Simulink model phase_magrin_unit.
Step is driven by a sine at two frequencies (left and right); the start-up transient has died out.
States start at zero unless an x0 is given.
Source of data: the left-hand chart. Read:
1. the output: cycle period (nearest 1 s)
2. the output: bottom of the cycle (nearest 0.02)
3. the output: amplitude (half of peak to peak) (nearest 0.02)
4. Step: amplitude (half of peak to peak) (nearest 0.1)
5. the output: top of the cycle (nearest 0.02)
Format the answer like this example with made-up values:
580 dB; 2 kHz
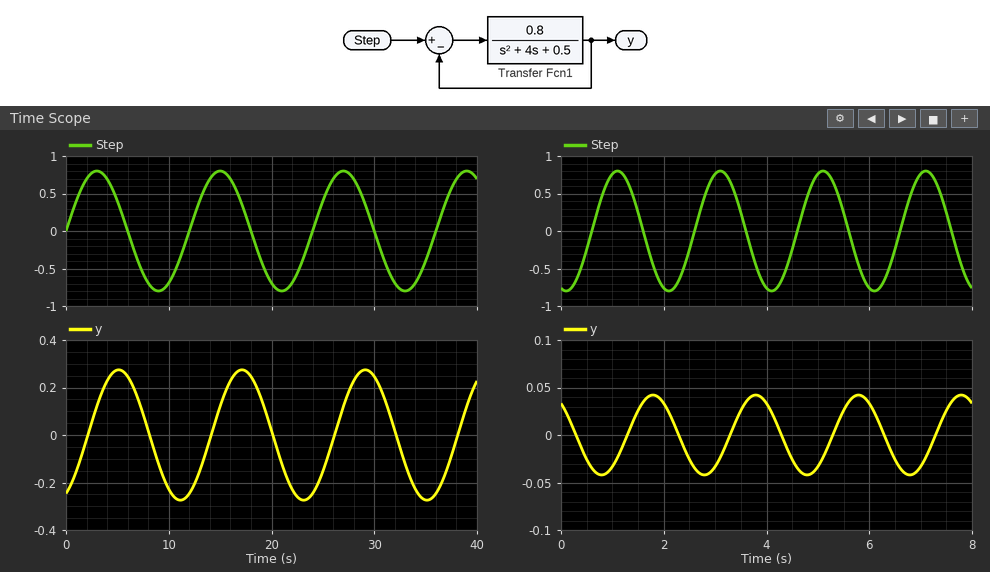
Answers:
12 s; -0.28; 0.28; 0.8; 0.28
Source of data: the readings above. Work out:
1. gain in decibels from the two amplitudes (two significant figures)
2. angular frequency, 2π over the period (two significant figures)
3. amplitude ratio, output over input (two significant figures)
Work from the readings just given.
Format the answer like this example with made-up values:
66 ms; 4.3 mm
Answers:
-9.1 dB; 0.52 rad/s; 0.35
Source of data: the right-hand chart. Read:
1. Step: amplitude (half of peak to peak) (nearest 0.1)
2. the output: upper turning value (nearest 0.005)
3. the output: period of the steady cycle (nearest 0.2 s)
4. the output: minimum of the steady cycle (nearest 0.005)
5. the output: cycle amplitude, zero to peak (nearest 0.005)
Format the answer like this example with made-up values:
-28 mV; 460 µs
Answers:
0.8; 0.040; 2.0 s; -0.040; 0.040
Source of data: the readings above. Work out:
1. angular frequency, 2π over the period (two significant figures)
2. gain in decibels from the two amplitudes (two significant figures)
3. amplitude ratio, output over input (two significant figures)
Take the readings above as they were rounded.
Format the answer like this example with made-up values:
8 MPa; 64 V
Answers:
3.1 rad/s; -26 dB; 0.050
